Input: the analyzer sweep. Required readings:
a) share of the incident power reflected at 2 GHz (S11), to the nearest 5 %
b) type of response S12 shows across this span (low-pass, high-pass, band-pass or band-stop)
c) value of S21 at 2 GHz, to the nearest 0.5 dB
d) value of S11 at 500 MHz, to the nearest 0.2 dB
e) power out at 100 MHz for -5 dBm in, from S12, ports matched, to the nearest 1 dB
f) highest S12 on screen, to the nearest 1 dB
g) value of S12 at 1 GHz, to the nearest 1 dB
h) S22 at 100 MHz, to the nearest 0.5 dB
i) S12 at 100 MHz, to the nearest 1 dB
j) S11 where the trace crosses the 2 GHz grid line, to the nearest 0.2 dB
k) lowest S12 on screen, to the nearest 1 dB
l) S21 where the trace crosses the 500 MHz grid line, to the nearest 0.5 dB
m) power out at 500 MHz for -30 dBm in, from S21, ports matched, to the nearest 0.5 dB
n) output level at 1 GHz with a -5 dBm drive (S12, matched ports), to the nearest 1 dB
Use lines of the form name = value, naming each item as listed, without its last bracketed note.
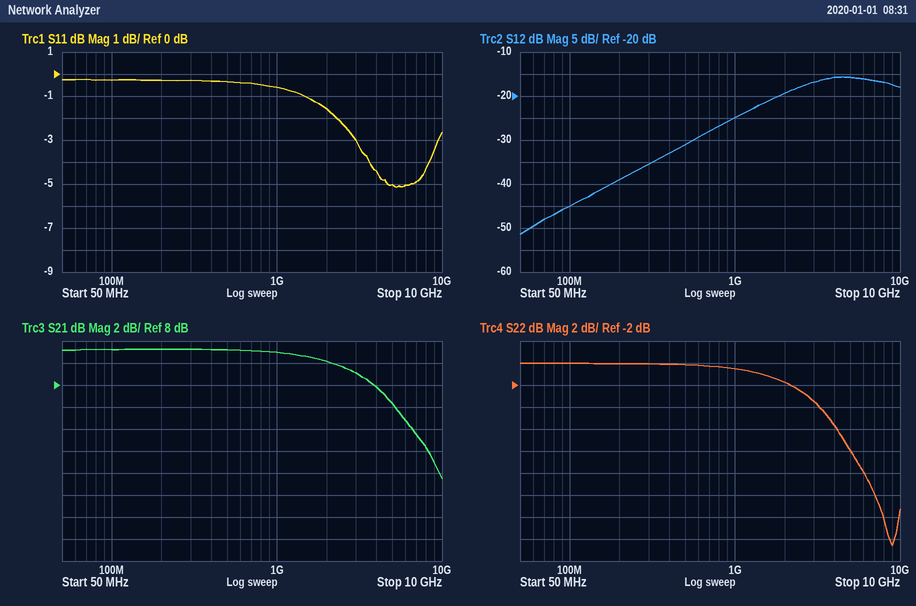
share of the incident power reflected at 2 GHz (S11), to the nearest 5 % = 70 %
type of response S12 shows across this span = high-pass
value of S21 at 2 GHz, to the nearest 0.5 dB = 10.0 dB
value of S11 at 500 MHz, to the nearest 0.2 dB = -0.4 dB
power out at 100 MHz for -5 dBm in, from S12, ports matched, to the nearest 1 dB = -50 dBm
highest S12 on screen, to the nearest 1 dB = -16 dB
value of S12 at 1 GHz, to the nearest 1 dB = -25 dB
S22 at 100 MHz, to the nearest 0.5 dB = 0.0 dB
S12 at 100 MHz, to the nearest 1 dB = -45 dB
S11 where the trace crosses the 2 GHz grid line, to the nearest 0.2 dB = -1.6 dB
lowest S12 on screen, to the nearest 1 dB = -51 dB
S21 where the trace crosses the 500 MHz grid line, to the nearest 0.5 dB = 11.0 dB
power out at 500 MHz for -30 dBm in, from S21, ports matched, to the nearest 0.5 dB = -19.0 dBm
output level at 1 GHz with a -5 dBm drive (S12, matched ports), to the nearest 1 dB = -30 dBm
